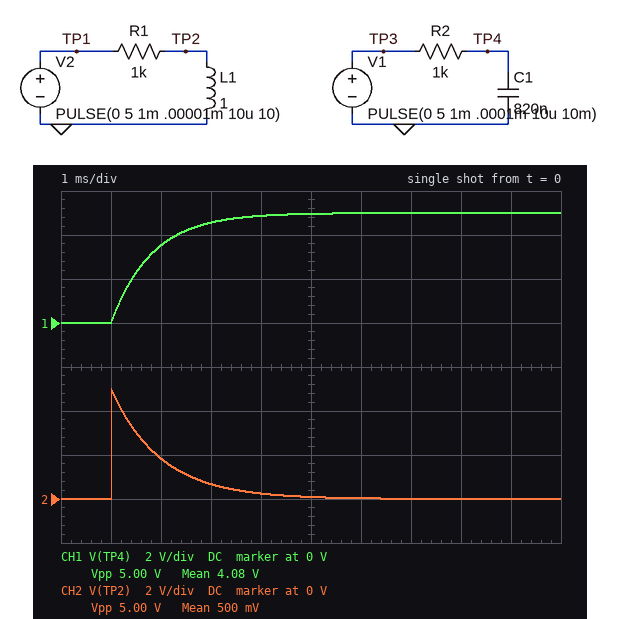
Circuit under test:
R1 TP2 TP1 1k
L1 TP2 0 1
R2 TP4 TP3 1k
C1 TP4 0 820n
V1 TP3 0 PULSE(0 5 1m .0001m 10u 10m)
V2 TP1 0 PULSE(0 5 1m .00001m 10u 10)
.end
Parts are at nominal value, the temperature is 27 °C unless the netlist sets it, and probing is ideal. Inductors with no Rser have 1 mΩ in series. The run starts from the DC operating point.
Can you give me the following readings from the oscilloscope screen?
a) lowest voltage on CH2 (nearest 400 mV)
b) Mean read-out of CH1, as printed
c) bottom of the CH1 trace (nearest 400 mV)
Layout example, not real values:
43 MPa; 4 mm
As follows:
0 V; 4.08 V; 0 V
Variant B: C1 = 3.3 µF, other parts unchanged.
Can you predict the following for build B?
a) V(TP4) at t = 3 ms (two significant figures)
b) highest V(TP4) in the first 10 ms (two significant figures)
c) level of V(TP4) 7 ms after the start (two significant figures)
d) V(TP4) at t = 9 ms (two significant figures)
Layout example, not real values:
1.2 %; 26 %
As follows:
2.3 V; 4.7 V; 4.2 V; 4.6 V
